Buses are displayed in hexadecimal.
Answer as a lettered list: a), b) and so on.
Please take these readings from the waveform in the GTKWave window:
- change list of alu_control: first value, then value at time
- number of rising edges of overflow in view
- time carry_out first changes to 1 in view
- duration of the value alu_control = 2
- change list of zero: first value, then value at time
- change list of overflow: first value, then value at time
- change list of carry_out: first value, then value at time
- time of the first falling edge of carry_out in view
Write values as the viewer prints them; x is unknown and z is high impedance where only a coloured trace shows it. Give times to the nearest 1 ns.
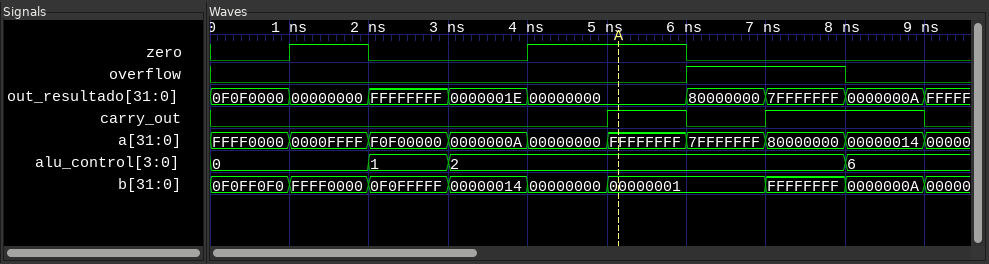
a) 0, 1 at 2 ns, 2 at 3 ns, 6 at 8 ns
b) 1
c) 5 ns
d) 5 ns
e) 0, 1 at 1 ns, 0 at 2 ns, 1 at 4 ns, 0 at 6 ns
f) 0, 1 at 6 ns, 0 at 8 ns
g) 0, 1 at 5 ns, 0 at 6 ns, 1 at 7 ns, 0 at 9 ns
h) 6 ns
